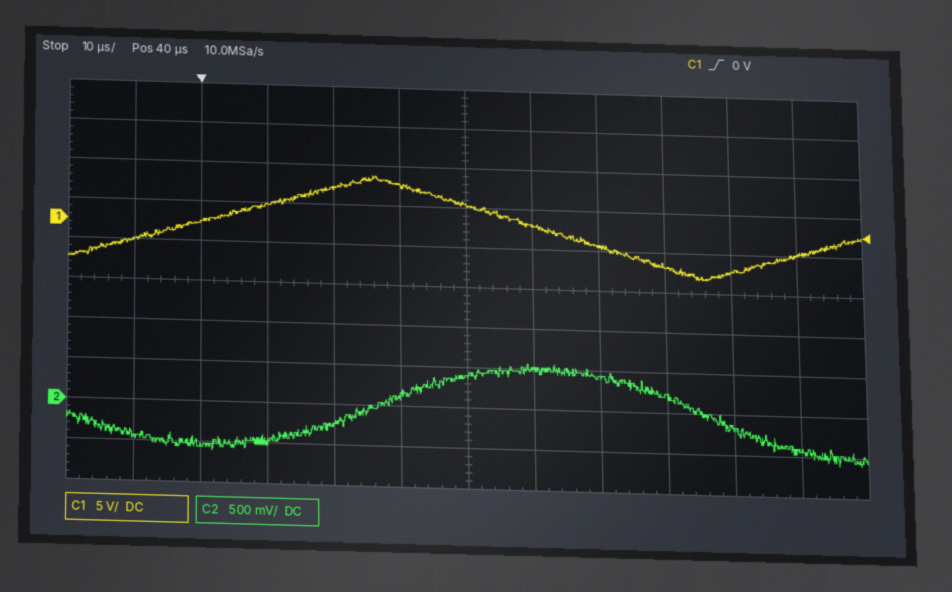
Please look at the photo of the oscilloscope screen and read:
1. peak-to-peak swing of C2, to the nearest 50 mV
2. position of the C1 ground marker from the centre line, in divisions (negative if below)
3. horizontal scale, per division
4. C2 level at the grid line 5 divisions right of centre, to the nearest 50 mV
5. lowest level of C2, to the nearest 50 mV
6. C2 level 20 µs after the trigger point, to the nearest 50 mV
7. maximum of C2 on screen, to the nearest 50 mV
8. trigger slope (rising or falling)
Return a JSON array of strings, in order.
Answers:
["1.15 V", "+1.5 div", "10 µs", "-400 mV", "-600 mV", "-250 mV", "550 mV", "rising"]
